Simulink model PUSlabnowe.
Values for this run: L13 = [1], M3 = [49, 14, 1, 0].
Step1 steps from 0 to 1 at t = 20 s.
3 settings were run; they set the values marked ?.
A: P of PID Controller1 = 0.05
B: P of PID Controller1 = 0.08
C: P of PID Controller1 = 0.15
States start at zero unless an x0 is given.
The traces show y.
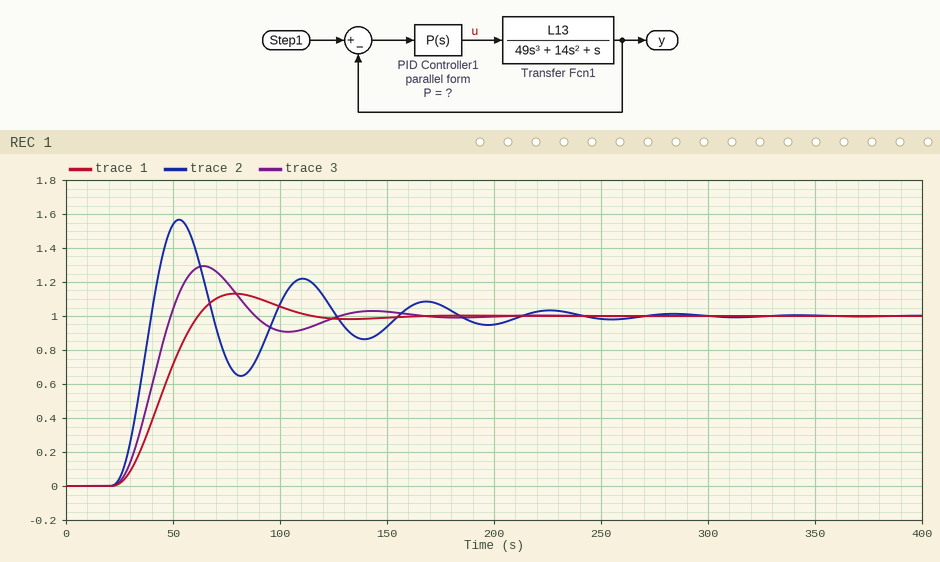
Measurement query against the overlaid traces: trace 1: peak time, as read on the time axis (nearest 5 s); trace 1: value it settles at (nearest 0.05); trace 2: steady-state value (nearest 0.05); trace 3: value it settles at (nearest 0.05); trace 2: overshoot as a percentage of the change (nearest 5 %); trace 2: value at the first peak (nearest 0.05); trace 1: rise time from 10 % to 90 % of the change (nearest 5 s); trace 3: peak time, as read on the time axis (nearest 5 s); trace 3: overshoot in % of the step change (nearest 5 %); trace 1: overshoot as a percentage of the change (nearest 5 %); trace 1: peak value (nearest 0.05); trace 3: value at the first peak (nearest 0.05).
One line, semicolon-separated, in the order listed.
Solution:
80 s; 1.00; 1.00; 1.00; 55 %; 1.55; 25 s; 65 s; 30 %; 15 %; 1.15; 1.30
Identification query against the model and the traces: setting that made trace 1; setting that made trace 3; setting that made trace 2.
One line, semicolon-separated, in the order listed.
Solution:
A; B; C
